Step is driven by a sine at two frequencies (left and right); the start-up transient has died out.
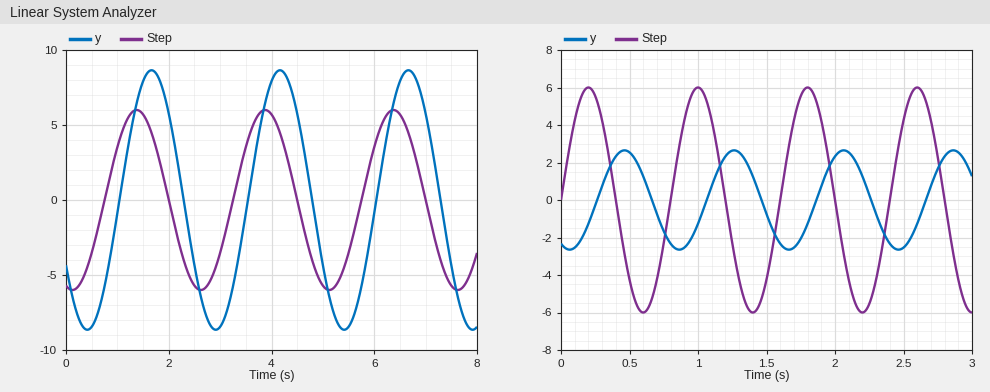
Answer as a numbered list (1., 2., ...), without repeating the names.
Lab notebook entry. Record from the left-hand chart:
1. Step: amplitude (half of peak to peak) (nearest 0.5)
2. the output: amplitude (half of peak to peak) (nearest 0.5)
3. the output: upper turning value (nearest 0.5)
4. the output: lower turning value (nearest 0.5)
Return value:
1. 6.0
2. 8.5
3. 8.5
4. -8.5
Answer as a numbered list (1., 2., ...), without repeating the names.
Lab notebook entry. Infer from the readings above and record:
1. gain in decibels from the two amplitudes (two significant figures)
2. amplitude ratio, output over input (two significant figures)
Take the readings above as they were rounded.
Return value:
1. 3.0 dB
2. 1.4
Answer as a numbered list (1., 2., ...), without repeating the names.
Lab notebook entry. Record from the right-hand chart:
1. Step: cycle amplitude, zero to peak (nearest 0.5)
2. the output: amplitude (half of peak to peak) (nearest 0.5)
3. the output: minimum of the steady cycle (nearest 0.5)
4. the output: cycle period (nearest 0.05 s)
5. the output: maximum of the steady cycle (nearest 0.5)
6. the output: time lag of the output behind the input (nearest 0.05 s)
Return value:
1. 6.0
2. 2.5
3. -2.5
4. 0.80 s
5. 2.5
6. 0.25 s
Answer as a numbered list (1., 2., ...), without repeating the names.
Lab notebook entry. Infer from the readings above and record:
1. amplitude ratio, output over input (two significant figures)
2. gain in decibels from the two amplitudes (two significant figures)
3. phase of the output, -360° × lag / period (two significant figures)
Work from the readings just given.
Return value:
1. 0.42
2. -7.6 dB
3. -110°
